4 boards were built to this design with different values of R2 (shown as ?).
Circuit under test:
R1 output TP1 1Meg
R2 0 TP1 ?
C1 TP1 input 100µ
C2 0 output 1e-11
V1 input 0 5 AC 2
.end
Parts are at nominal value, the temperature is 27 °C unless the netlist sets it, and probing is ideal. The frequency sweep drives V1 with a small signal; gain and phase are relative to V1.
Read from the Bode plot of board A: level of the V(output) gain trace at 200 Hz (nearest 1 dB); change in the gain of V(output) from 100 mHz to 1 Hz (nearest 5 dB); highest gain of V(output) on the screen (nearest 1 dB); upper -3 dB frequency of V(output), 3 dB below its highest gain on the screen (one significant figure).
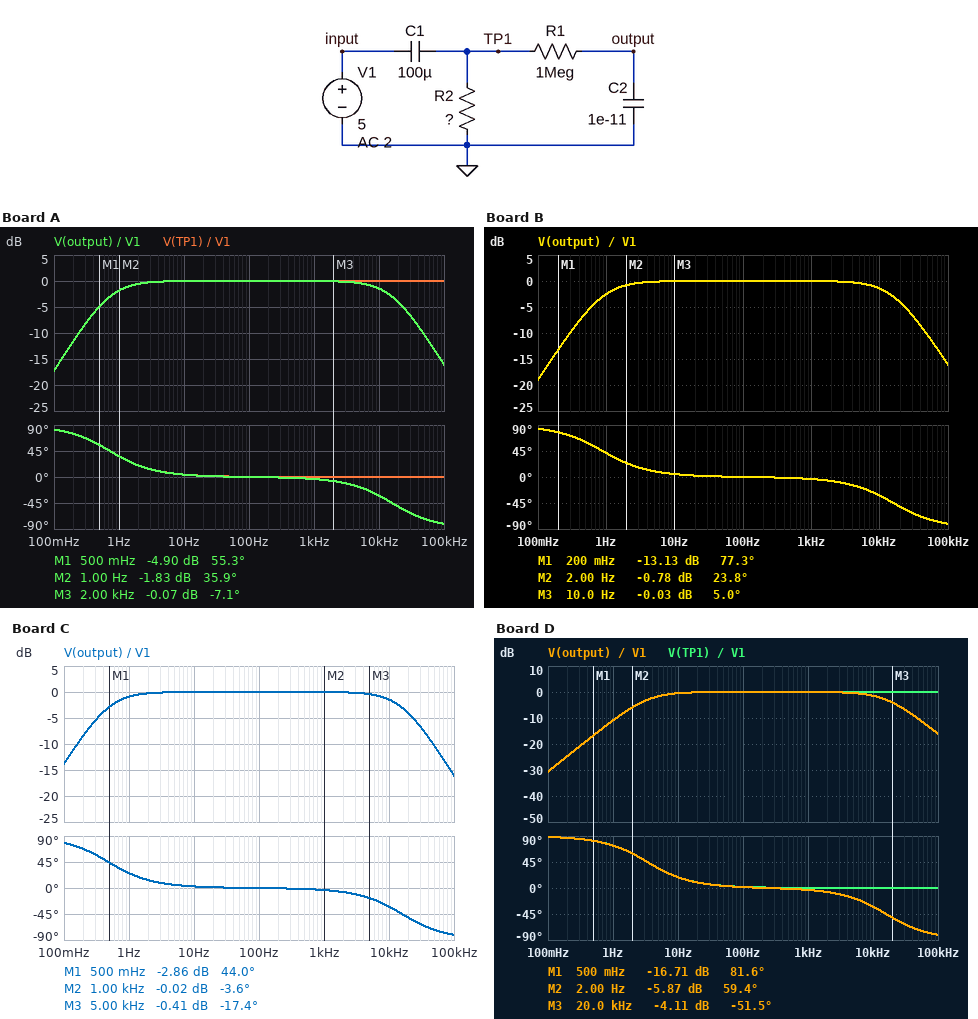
0 dB
15 dB
0 dB
20 kHz
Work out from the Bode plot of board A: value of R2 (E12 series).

2.2 kΩ
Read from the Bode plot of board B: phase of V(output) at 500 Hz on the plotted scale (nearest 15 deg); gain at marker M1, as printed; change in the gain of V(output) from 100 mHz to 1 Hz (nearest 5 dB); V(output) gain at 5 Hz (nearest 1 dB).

0 deg
-13.13 dB
15 dB
0 dB
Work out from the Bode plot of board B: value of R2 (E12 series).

1.8 kΩ
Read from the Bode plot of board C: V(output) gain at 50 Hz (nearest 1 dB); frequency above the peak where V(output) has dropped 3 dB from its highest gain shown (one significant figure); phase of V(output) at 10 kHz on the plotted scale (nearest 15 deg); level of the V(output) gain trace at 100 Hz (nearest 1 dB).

0 dB
20 kHz
-30 deg
0 dB
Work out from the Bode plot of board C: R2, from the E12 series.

3.3 kΩ
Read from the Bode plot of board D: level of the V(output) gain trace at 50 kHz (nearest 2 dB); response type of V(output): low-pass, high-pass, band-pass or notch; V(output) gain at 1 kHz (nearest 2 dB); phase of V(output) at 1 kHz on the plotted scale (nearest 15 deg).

-10 dB
band-pass
0 dB
0 deg
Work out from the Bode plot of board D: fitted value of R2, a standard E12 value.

470 Ω
